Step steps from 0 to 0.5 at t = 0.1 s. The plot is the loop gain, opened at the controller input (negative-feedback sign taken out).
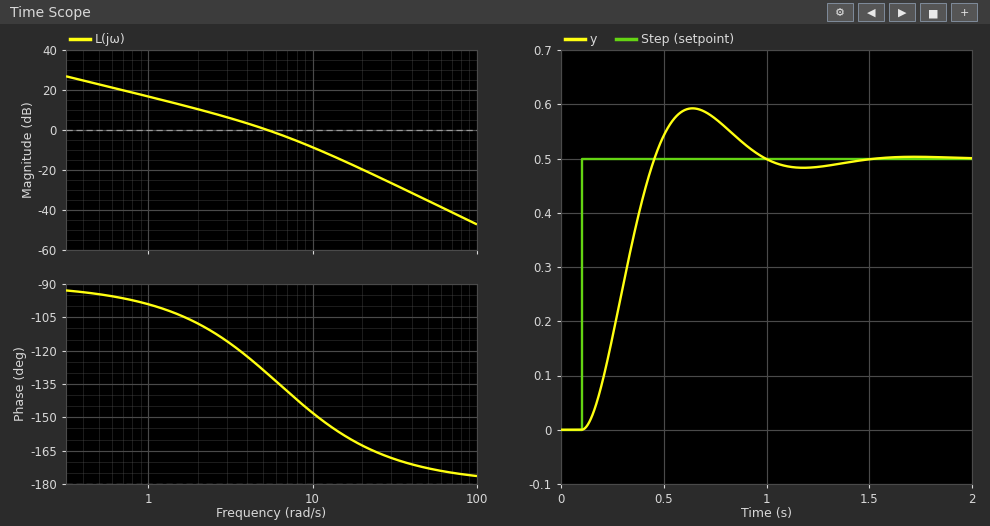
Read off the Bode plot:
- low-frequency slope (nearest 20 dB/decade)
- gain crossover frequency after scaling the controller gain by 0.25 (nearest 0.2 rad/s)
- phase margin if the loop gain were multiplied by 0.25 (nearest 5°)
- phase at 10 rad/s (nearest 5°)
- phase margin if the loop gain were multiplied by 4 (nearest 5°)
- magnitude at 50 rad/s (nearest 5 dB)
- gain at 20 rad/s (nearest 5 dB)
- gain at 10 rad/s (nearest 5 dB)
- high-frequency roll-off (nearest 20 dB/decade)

-20 dB/decade
1.6 rad/s
75°
-150°
25°
-35 dB
-20 dB
-10 dB
-40 dB/decade
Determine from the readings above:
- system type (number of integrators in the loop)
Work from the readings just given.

1
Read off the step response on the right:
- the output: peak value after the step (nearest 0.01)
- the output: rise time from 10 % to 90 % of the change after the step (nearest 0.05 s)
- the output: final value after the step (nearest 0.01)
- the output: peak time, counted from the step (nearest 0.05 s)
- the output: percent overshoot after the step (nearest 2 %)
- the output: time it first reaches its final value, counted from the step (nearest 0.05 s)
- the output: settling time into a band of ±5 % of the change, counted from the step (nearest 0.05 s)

0.59
0.25 s
0.50
0.55 s
18 %
0.35 s
0.80 s
